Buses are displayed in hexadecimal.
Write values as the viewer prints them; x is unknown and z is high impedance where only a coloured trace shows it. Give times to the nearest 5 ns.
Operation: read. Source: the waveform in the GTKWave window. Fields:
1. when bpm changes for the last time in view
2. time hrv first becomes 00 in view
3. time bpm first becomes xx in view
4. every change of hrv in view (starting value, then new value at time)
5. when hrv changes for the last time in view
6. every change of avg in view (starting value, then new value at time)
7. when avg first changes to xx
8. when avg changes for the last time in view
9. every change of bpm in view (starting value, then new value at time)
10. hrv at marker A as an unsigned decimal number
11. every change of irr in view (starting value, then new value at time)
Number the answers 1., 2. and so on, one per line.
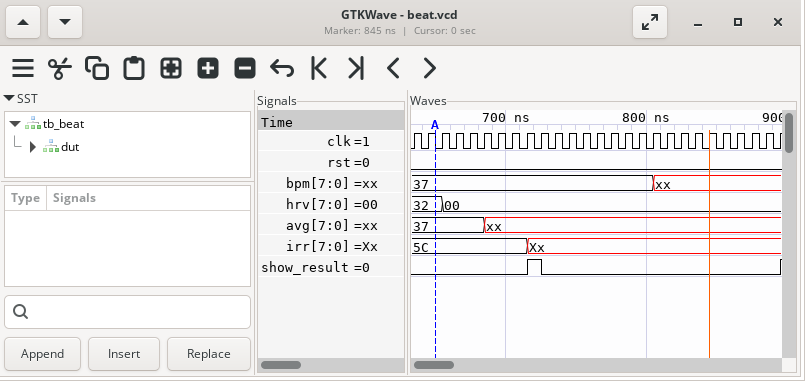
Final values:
1. 805 ns
2. 655 ns
3. 805 ns
4. 32, 00 at 655 ns
5. 655 ns
6. 37, xx at 685 ns
7. 685 ns
8. 685 ns
9. 37, xx at 805 ns
10. 50
11. 5C, Xx at 715 ns
